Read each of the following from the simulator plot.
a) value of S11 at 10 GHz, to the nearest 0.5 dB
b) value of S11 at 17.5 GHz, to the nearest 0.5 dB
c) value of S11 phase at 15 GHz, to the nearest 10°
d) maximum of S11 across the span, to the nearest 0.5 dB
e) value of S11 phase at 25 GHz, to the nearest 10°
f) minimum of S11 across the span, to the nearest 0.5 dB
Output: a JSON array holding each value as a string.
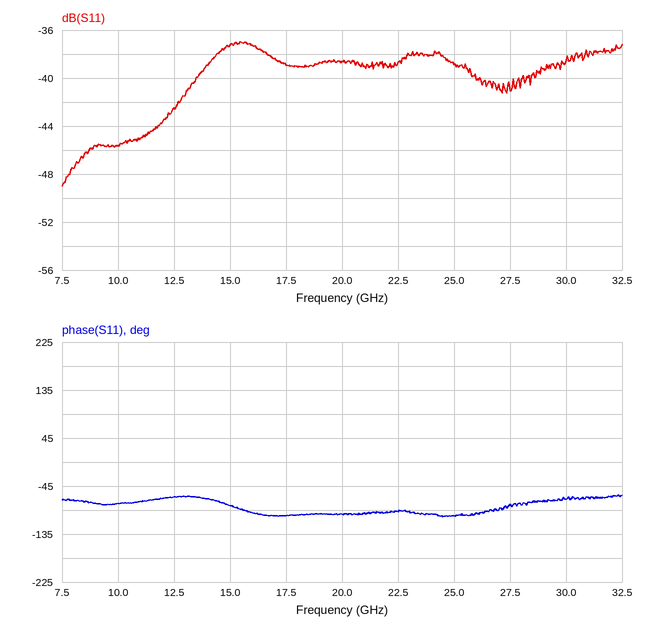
["-45.5 dB", "-39.0 dB", "-80°", "-37.0 dB", "-100°", "-49.0 dB"]
